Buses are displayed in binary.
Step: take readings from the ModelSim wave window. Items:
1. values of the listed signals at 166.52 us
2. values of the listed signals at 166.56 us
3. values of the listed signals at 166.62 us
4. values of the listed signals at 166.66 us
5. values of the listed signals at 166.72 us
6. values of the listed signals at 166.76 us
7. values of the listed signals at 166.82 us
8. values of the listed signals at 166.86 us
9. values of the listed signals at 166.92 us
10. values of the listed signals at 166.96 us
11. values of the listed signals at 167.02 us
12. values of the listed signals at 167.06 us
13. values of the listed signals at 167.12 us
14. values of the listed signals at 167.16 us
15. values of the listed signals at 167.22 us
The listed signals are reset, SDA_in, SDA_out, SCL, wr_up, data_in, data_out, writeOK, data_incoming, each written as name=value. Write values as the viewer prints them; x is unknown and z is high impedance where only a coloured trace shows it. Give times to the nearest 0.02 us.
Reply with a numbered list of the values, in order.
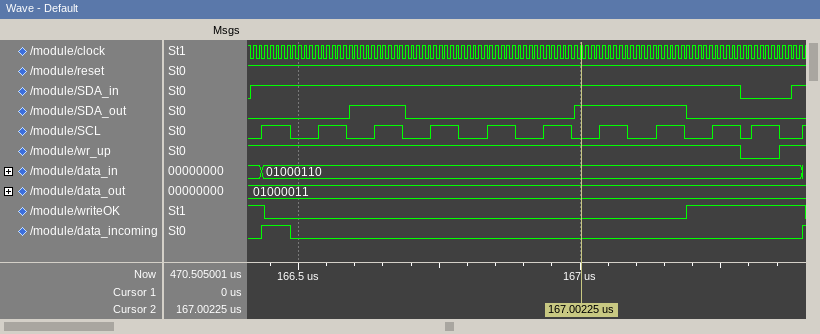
1. reset=1, SDA_in=1, SDA_out=0, SCL=0, wr_up=1, data_in=01000110, data_out=01000011, writeOK=0, data_incoming=0
2. reset=1, SDA_in=1, SDA_out=0, SCL=1, wr_up=1, data_in=01000110, data_out=01000011, writeOK=0, data_incoming=0
3. reset=1, SDA_in=1, SDA_out=1, SCL=0, wr_up=1, data_in=01000110, data_out=01000011, writeOK=0, data_incoming=0
4. reset=1, SDA_in=1, SDA_out=1, SCL=1, wr_up=1, data_in=01000110, data_out=01000011, writeOK=0, data_incoming=0
5. reset=1, SDA_in=1, SDA_out=0, SCL=0, wr_up=1, data_in=01000110, data_out=01000011, writeOK=0, data_incoming=0
6. reset=1, SDA_in=1, SDA_out=0, SCL=1, wr_up=1, data_in=01000110, data_out=01000011, writeOK=0, data_incoming=0
7. reset=1, SDA_in=1, SDA_out=0, SCL=0, wr_up=1, data_in=01000110, data_out=01000011, writeOK=0, data_incoming=0
8. reset=1, SDA_in=1, SDA_out=0, SCL=1, wr_up=1, data_in=01000110, data_out=01000011, writeOK=0, data_incoming=0
9. reset=1, SDA_in=1, SDA_out=0, SCL=0, wr_up=1, data_in=01000110, data_out=01000011, writeOK=0, data_incoming=0
10. reset=1, SDA_in=1, SDA_out=0, SCL=1, wr_up=1, data_in=01000110, data_out=01000011, writeOK=0, data_incoming=0
11. reset=1, SDA_in=1, SDA_out=1, SCL=0, wr_up=1, data_in=01000110, data_out=01000011, writeOK=0, data_incoming=0
12. reset=1, SDA_in=1, SDA_out=1, SCL=1, wr_up=1, data_in=01000110, data_out=01000011, writeOK=0, data_incoming=0
13. reset=1, SDA_in=1, SDA_out=1, SCL=0, wr_up=1, data_in=01000110, data_out=01000011, writeOK=0, data_incoming=0
14. reset=1, SDA_in=1, SDA_out=1, SCL=1, wr_up=1, data_in=01000110, data_out=01000011, writeOK=0, data_incoming=0
15. reset=1, SDA_in=1, SDA_out=0, SCL=0, wr_up=1, data_in=01000110, data_out=01000011, writeOK=1, data_incoming=0
